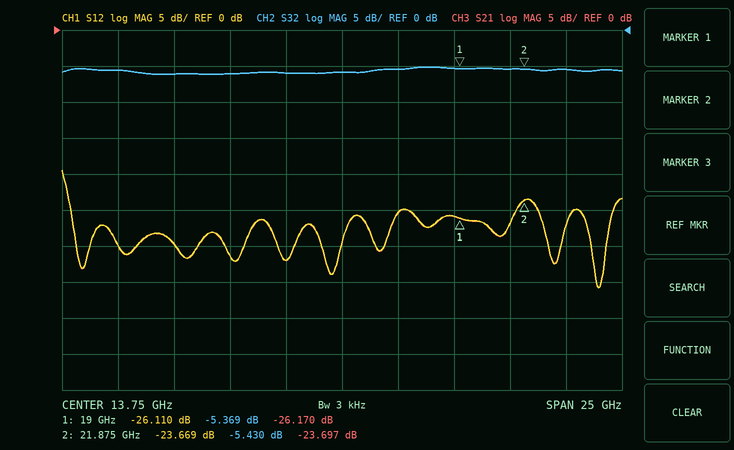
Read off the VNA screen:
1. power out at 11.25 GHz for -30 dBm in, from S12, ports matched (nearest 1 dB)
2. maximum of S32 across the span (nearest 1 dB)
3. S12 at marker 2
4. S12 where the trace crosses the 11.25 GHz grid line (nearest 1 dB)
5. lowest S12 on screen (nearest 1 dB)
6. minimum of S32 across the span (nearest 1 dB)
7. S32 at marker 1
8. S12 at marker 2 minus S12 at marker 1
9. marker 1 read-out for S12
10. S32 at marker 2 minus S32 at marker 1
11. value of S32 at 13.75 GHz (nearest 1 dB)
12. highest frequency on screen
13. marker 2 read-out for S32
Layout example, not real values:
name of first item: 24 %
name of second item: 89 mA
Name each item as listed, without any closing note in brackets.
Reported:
power out at 11.25 GHz for -30 dBm in, from S12, ports matched: -62 dBm
maximum of S32 across the span: -5 dB
S12 at marker 2: -23.669 dB
S12 where the trace crosses the 11.25 GHz grid line: -32 dB
lowest S12 on screen: -36 dB
minimum of S32 across the span: -6 dB
S32 at marker 1: -5.369 dB
S12 at marker 2 minus S12 at marker 1: 2.441 dB
marker 1 read-out for S12: -26.110 dB
S32 at marker 2 minus S32 at marker 1: -0.061 dB
value of S32 at 13.75 GHz: -6 dB
highest frequency on screen: 26.25 GHz
marker 2 read-out for S32: -5.430 dB
